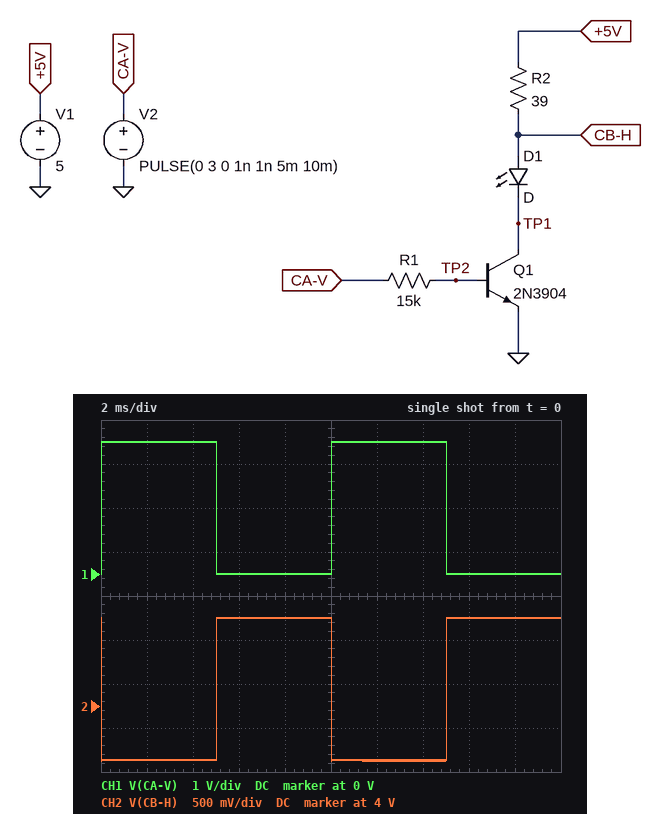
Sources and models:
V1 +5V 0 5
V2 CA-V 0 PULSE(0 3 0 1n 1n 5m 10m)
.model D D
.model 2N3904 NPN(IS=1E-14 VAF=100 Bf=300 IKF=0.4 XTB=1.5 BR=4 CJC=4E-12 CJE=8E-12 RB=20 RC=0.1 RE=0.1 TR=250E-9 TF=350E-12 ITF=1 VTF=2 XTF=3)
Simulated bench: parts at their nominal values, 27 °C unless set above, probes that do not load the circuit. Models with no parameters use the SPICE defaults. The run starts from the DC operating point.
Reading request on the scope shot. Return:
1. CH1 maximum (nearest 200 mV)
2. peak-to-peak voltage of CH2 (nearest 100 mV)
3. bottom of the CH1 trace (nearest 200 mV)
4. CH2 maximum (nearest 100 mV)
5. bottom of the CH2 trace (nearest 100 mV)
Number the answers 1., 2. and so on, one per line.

1. 3.0 V
2. 1.6 V
3. 0 V
4. 5.0 V
5. 3.4 V
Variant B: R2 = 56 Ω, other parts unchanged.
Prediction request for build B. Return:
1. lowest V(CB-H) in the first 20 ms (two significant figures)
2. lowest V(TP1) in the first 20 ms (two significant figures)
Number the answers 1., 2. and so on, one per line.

1. 2.7 V
2. 1.9 V
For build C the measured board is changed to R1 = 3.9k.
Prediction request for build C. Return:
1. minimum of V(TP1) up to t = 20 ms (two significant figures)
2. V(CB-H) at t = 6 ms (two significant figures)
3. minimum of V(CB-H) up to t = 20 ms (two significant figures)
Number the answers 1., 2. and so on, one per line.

1. 170 mV
2. 5.0 V
3. 940 mV
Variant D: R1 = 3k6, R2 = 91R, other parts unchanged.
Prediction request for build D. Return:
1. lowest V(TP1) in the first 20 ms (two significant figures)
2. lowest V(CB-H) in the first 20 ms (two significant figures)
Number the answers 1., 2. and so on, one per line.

1. 97 mV
2. 850 mV
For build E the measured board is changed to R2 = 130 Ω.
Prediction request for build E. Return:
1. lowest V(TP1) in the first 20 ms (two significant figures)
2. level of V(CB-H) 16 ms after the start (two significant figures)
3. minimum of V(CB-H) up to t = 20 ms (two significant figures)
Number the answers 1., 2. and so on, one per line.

1. 150 mV
2. 5.0 V
3. 890 mV
